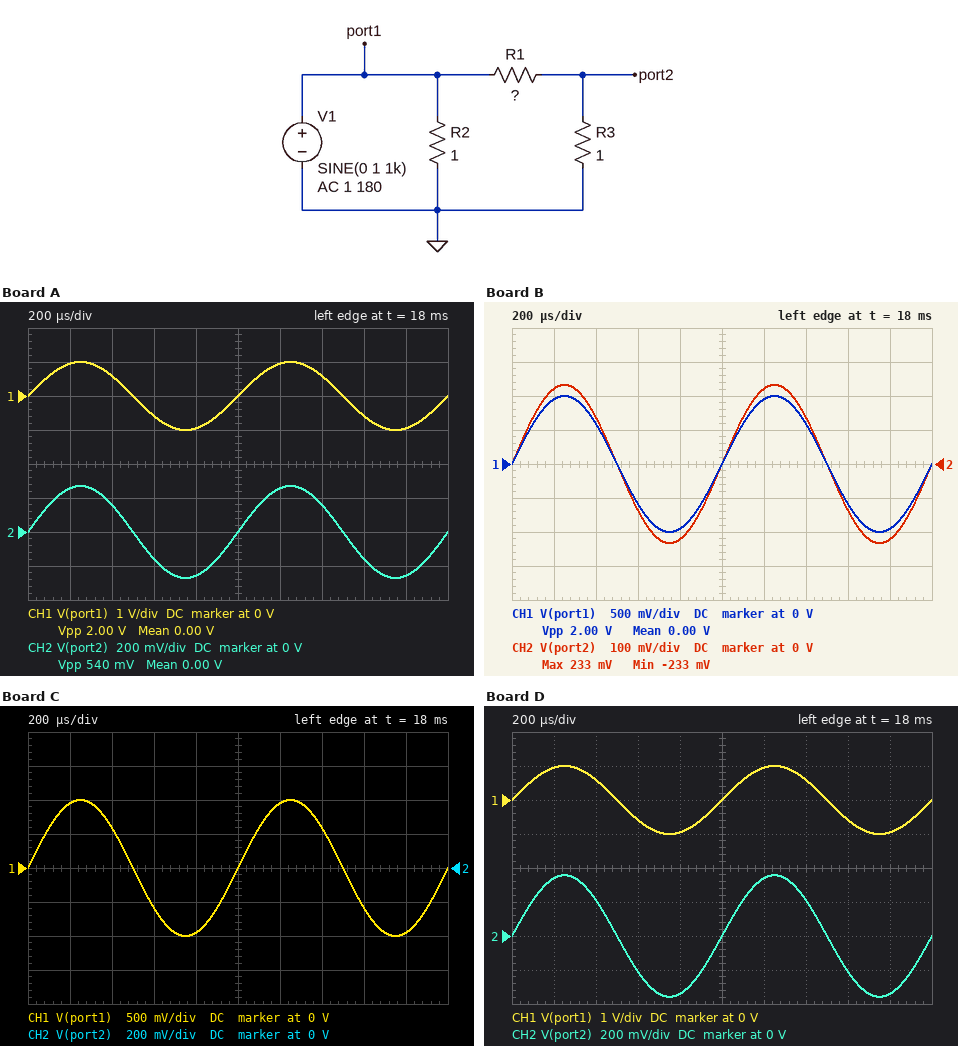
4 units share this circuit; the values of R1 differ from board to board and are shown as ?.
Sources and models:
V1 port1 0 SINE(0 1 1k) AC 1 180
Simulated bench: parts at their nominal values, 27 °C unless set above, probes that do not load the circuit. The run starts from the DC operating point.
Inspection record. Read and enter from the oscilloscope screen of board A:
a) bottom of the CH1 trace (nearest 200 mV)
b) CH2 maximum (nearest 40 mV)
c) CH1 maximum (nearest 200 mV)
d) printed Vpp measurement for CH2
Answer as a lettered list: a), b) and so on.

a) -1.0 V
b) 280 mV
c) 1.0 V
d) 540 mV
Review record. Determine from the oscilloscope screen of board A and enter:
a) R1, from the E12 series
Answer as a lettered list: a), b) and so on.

a) 2.7 Ω
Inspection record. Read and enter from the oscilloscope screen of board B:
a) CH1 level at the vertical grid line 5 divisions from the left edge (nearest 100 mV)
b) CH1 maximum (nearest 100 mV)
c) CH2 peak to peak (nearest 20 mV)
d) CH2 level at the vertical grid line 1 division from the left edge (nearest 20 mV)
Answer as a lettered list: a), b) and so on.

a) 0 V
b) 1.0 V
c) 460 mV
d) 220 mV
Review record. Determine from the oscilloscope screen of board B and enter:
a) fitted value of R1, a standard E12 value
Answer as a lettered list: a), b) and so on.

a) 3.3 Ω
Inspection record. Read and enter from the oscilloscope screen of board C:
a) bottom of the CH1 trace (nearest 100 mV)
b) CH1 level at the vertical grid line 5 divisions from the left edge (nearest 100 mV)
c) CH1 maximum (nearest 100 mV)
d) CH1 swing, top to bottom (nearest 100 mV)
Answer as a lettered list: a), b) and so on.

a) -1.0 V
b) 0 V
c) 1.0 V
d) 2.0 V
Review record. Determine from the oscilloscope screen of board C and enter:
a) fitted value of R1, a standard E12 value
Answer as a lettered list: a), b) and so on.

a) 1.5 Ω
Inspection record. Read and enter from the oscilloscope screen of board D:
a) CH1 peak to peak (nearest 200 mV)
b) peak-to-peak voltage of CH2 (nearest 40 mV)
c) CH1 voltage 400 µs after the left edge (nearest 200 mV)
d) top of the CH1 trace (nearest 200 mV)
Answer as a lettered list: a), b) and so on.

a) 2.0 V
b) 720 mV
c) 600 mV
d) 1.0 V
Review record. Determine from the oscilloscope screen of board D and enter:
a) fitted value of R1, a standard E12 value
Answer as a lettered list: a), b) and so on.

a) 1.8 Ω
